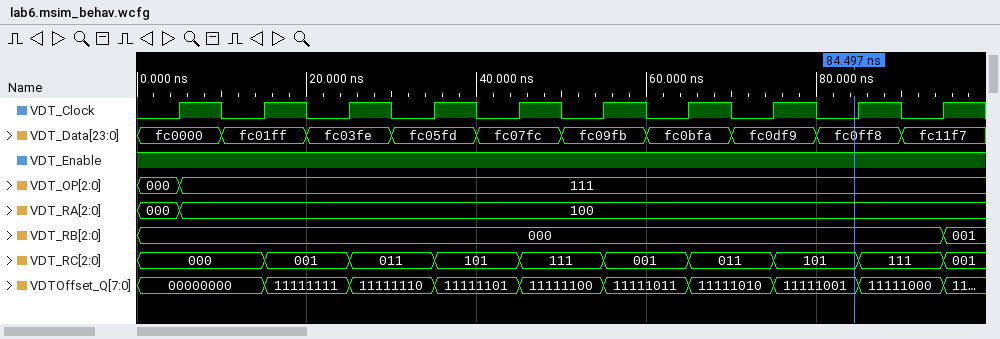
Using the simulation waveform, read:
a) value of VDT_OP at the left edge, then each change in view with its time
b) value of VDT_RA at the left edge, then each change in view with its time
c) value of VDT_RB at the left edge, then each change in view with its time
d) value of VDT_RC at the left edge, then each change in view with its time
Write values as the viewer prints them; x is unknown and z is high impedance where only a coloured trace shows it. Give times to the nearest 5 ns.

000, 111 at 5 ns
000, 100 at 5 ns
000, 001 at 95 ns
000, 001 at 15 ns, 011 at 25 ns, 101 at 35 ns, 111 at 45 ns, 001 at 55 ns, 011 at 65 ns, 101 at 75 ns, 111 at 85 ns, 001 at 95 ns
